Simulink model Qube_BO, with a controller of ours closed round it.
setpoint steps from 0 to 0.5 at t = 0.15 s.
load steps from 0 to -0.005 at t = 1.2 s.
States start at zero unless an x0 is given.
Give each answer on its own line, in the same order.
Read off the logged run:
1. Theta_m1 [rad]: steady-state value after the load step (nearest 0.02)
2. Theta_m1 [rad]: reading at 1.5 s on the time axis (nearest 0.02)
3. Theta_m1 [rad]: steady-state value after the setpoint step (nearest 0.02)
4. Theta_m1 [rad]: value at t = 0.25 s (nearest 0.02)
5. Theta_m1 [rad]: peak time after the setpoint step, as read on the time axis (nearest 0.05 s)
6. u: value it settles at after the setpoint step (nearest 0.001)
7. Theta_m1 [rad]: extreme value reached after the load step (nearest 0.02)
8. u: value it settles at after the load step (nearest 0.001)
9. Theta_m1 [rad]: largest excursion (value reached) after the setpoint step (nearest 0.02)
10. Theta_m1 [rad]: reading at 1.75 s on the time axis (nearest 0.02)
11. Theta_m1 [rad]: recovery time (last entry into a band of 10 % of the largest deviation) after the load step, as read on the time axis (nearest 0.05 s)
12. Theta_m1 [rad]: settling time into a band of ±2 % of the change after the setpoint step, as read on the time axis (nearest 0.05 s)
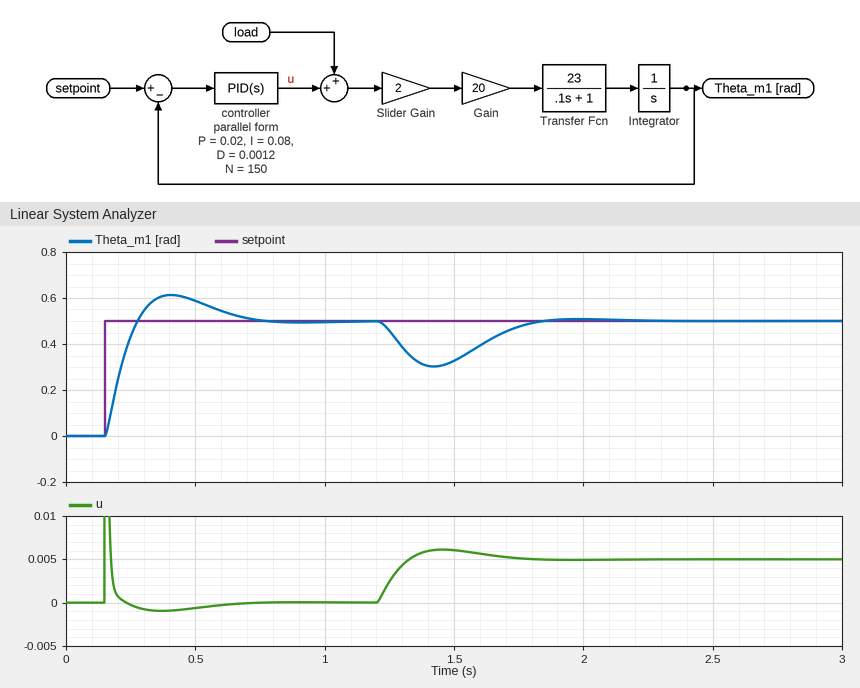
0.50
0.32
0.50
0.44
0.40 s
0.000
0.30
0.005
0.62
0.48
1.75 s
0.70 s
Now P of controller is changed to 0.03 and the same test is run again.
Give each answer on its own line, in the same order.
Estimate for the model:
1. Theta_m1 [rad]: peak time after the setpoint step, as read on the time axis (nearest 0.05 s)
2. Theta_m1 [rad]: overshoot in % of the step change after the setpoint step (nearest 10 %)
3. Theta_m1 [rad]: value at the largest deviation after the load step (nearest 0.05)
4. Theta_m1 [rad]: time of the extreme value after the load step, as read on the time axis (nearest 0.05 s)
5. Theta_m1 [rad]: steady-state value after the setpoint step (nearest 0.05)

0.35 s
20 %
0.35
1.40 s
0.50
